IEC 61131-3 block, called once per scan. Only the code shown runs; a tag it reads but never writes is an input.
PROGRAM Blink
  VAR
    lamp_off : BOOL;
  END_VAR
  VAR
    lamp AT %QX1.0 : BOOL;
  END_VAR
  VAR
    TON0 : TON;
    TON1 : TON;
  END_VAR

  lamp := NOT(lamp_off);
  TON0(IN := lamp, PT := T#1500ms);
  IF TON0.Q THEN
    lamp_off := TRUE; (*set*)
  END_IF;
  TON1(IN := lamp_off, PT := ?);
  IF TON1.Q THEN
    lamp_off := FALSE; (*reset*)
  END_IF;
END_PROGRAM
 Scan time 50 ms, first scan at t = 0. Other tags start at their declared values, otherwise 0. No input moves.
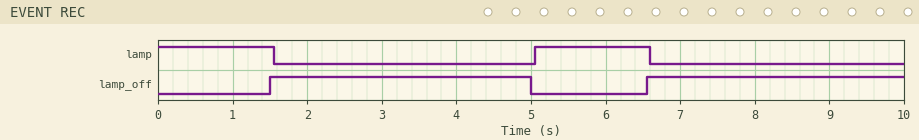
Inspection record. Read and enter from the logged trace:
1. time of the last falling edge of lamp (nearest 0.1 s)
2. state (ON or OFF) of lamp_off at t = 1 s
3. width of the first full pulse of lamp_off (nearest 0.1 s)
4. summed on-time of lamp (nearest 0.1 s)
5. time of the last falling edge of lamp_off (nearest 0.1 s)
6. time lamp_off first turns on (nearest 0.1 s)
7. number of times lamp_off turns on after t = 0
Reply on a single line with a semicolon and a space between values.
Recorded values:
6.6 s; OFF; 3.5 s; 3.1 s; 5.0 s; 1.5 s; 2
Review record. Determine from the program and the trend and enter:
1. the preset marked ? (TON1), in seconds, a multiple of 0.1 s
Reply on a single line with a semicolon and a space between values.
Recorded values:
3.5 s
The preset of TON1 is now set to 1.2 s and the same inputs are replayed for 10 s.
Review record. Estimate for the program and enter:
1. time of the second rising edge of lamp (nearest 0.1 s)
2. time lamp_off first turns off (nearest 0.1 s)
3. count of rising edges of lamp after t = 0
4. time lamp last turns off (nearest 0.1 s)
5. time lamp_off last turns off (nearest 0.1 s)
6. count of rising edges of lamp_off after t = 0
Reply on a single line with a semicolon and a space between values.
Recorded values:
5.5 s; 2.7 s; 3; 9.8 s; 8.2 s; 4
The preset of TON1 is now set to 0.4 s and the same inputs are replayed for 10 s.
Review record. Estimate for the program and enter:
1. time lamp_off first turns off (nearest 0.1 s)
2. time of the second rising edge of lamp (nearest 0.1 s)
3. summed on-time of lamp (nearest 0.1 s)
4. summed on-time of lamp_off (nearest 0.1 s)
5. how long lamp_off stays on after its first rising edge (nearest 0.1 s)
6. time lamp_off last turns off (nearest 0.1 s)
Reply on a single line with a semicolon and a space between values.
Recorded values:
1.9 s; 3.9 s; 8.0 s; 2.0 s; 0.4 s; 9.7 s
